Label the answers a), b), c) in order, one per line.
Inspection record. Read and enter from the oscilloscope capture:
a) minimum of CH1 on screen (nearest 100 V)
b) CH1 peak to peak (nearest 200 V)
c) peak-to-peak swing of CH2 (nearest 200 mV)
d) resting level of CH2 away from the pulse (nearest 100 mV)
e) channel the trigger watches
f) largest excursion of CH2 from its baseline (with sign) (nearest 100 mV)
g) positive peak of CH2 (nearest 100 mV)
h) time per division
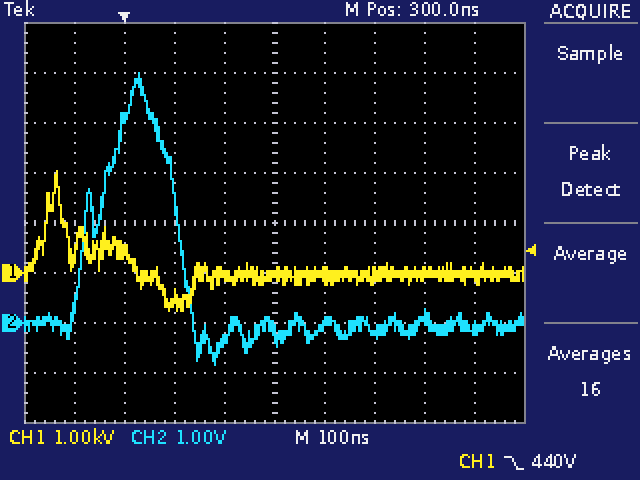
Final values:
a) -800 V
b) 2.8 kV
c) 5.8 V
d) 0.0 V
e) CH1
f) +5.0 V
g) 5.0 V
h) 100 ns
